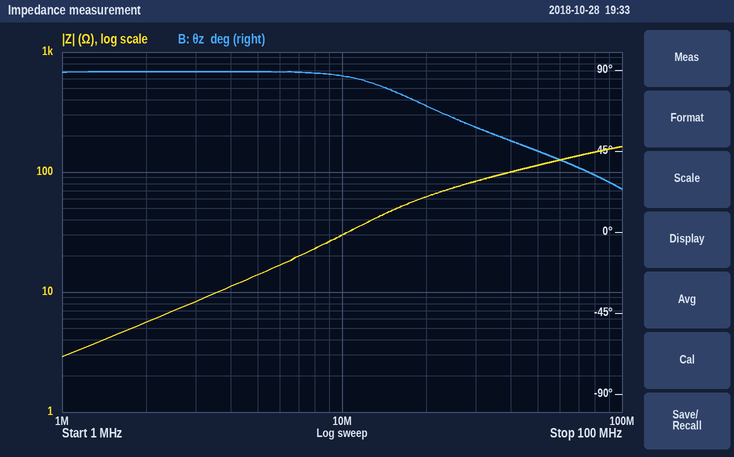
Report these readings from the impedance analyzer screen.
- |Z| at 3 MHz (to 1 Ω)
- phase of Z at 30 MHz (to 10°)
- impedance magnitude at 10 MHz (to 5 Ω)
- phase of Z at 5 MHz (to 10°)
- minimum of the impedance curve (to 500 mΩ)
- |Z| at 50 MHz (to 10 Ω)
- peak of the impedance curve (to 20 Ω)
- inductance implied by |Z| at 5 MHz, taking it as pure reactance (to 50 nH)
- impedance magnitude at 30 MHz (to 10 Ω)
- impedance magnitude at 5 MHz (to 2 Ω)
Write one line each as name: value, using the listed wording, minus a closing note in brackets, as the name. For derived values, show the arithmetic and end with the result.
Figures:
|Z| at 3 MHz: 8 Ω
phase of Z at 30 MHz: 60°
impedance magnitude at 10 MHz: 30 Ω
phase of Z at 5 MHz: 90°
minimum of the impedance curve: 3.0 Ω
|Z| at 50 MHz: 110 Ω
peak of the impedance curve: 160 Ω
inductance implied by |Z| at 5 MHz, taking it as pure reactance: L = 14 Ω/(2π × 5 MHz) ≈ 446 nH, so 450 nH to the nearest 50 nH
impedance magnitude at 30 MHz: 80 Ω
impedance magnitude at 5 MHz: 14 Ω
